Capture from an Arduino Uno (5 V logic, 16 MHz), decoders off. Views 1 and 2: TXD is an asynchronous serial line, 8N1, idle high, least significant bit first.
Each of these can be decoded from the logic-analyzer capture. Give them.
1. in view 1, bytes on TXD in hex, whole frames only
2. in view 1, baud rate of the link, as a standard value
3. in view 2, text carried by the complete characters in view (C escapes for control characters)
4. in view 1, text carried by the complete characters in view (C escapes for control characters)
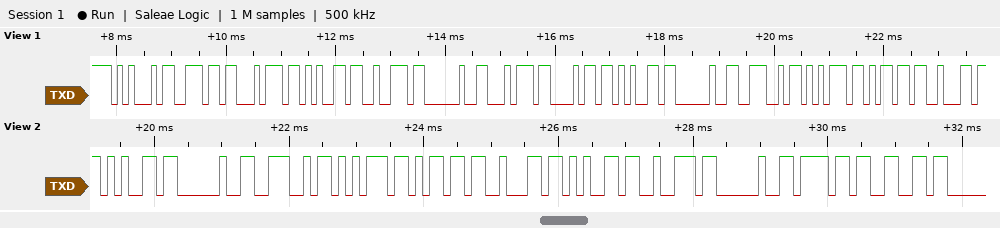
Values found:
45 6E 74 65 72 20 74 68 65 20 4E 75 6D 62
9600 baud
"e Number of"
"Enter the Numb"
